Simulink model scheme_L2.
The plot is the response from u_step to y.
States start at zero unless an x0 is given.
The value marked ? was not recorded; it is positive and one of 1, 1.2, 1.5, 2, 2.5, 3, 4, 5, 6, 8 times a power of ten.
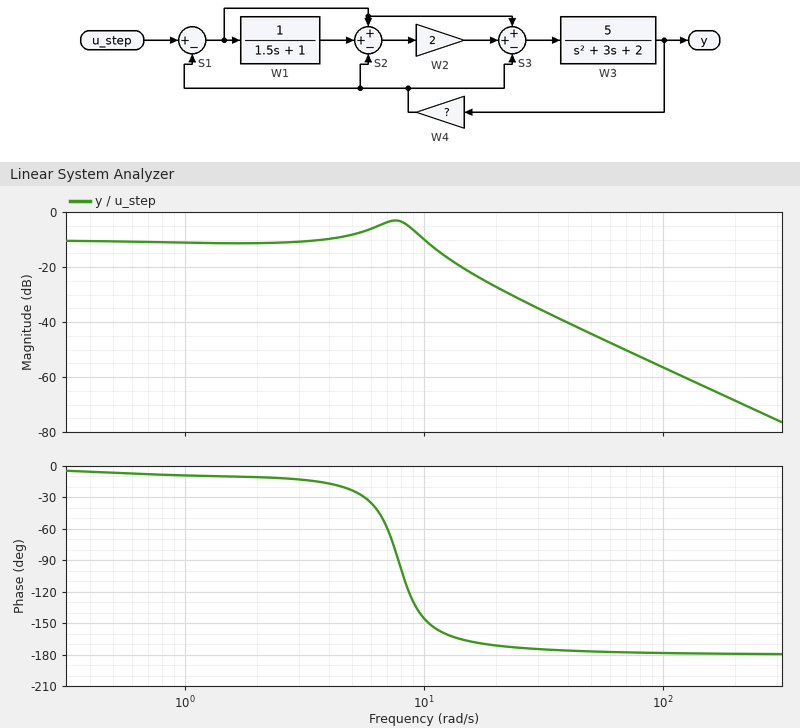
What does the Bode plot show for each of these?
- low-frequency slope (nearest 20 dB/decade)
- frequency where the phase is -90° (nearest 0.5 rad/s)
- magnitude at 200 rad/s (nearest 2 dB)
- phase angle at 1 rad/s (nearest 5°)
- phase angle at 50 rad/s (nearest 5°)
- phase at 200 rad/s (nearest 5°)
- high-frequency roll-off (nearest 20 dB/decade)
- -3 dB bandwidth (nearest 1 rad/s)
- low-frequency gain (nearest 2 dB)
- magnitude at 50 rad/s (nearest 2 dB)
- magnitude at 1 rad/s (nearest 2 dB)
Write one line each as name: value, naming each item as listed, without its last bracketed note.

low-frequency slope: 0 dB/decade
frequency where the phase is -90°: 8.0 rad/s
magnitude at 200 rad/s: -68 dB
phase angle at 1 rad/s: -10°
phase angle at 50 rad/s: -175°
phase at 200 rad/s: -180°
high-frequency roll-off: -40 dB/decade
-3 dB bandwidth: 11 rad/s
low-frequency gain: -10 dB
magnitude at 50 rad/s: -44 dB
magnitude at 1 rad/s: -12 dB
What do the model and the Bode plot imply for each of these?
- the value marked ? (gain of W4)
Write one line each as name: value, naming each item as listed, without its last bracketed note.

the value marked ?: 2
